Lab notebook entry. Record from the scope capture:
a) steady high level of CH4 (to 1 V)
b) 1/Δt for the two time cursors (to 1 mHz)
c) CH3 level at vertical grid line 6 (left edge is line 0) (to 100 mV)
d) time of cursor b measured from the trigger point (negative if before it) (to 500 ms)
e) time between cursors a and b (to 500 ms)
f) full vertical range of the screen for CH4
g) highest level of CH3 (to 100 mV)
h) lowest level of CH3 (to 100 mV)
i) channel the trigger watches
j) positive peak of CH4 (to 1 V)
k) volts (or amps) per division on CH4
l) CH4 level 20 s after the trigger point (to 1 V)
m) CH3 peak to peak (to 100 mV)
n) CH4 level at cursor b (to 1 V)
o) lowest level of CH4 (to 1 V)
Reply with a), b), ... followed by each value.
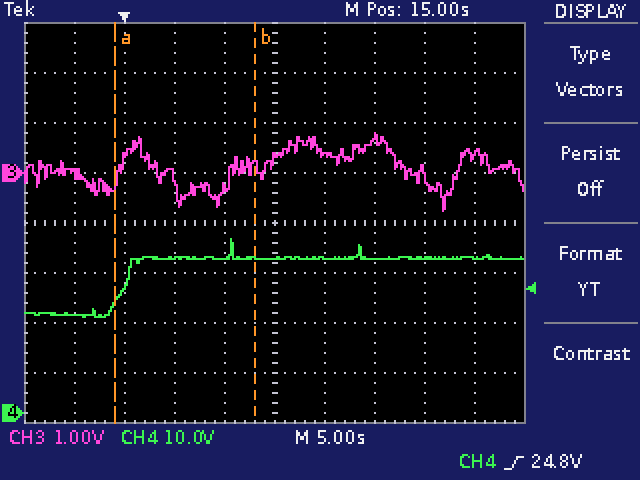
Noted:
a) 31 V
b) 71 mHz
c) 400 mV
d) +13.0 s
e) 14.0 s
f) 80 V
g) 800 mV
h) -800 mV
i) CH4
j) 35 V
k) 10 V
l) 31 V
m) 1.6 V
n) 31 V
o) 19 V
